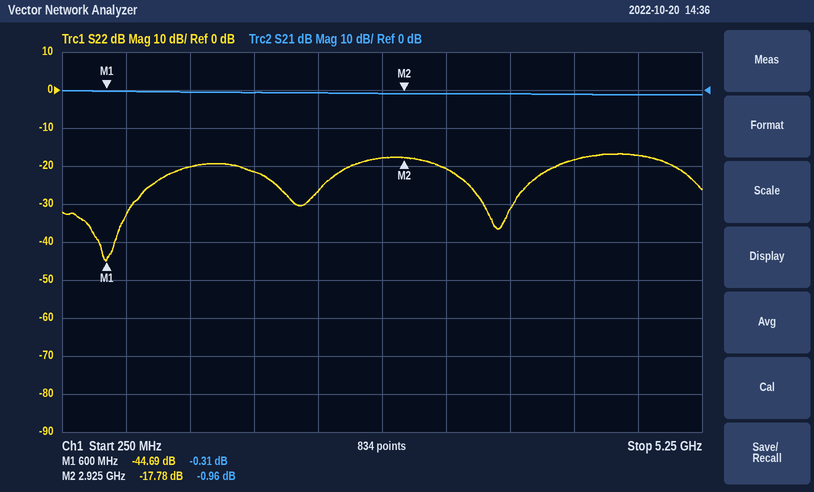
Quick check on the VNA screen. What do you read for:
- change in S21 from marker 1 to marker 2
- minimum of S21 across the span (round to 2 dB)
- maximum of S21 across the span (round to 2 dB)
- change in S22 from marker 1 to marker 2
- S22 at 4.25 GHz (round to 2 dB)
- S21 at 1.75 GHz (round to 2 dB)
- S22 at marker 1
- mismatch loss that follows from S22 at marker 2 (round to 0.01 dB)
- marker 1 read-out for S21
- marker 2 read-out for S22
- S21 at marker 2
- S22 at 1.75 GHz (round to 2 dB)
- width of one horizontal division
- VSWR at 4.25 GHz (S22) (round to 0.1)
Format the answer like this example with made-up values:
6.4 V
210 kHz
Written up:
-0.65 dB
-2 dB
0 dB
26.91 dB
-18 dB
0 dB
-44.69 dB
0.07 dB
-0.31 dB
-17.78 dB
-0.96 dB
-22 dB
500 MHz
1.3
